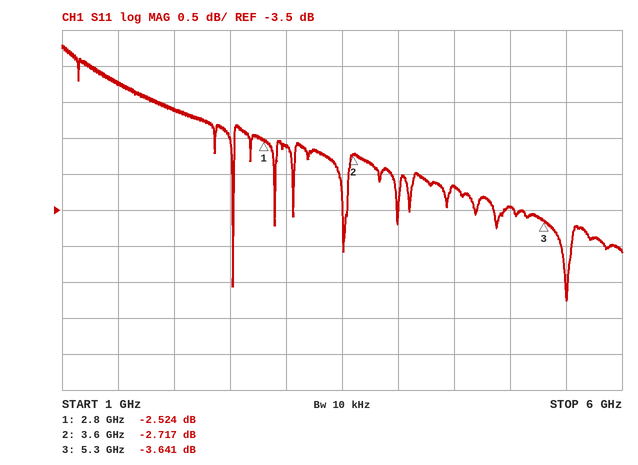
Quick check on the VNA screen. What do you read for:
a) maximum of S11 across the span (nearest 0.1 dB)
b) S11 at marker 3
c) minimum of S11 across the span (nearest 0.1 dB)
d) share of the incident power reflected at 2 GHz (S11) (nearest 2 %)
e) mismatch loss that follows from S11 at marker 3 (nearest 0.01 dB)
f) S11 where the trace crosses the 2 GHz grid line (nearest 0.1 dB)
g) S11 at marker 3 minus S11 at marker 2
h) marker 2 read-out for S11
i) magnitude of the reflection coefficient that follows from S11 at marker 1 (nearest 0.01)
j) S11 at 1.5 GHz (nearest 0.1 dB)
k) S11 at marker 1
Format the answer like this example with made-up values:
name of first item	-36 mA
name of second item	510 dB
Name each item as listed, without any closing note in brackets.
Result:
maximum of S11 across the span	-1.2 dB
S11 at marker 3	-3.641 dB
minimum of S11 across the span	-4.8 dB
share of the incident power reflected at 2 GHz (S11)	62 %
mismatch loss that follows from S11 at marker 3	2.46 dB
S11 where the trace crosses the 2 GHz grid line	-2.1 dB
S11 at marker 3 minus S11 at marker 2	-0.924 dB
marker 2 read-out for S11	-2.717 dB
magnitude of the reflection coefficient that follows from S11 at marker 1	0.75
S11 at 1.5 GHz	-1.7 dB
S11 at marker 1	-2.524 dB
